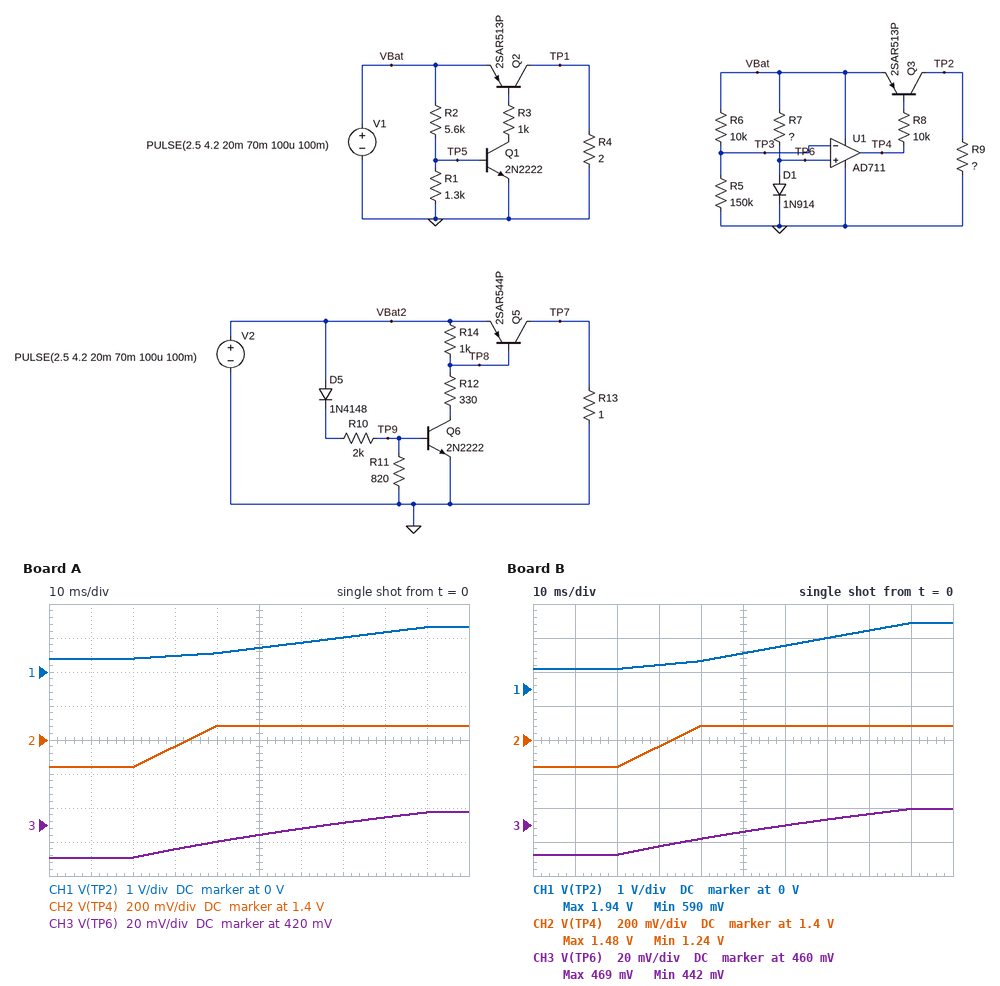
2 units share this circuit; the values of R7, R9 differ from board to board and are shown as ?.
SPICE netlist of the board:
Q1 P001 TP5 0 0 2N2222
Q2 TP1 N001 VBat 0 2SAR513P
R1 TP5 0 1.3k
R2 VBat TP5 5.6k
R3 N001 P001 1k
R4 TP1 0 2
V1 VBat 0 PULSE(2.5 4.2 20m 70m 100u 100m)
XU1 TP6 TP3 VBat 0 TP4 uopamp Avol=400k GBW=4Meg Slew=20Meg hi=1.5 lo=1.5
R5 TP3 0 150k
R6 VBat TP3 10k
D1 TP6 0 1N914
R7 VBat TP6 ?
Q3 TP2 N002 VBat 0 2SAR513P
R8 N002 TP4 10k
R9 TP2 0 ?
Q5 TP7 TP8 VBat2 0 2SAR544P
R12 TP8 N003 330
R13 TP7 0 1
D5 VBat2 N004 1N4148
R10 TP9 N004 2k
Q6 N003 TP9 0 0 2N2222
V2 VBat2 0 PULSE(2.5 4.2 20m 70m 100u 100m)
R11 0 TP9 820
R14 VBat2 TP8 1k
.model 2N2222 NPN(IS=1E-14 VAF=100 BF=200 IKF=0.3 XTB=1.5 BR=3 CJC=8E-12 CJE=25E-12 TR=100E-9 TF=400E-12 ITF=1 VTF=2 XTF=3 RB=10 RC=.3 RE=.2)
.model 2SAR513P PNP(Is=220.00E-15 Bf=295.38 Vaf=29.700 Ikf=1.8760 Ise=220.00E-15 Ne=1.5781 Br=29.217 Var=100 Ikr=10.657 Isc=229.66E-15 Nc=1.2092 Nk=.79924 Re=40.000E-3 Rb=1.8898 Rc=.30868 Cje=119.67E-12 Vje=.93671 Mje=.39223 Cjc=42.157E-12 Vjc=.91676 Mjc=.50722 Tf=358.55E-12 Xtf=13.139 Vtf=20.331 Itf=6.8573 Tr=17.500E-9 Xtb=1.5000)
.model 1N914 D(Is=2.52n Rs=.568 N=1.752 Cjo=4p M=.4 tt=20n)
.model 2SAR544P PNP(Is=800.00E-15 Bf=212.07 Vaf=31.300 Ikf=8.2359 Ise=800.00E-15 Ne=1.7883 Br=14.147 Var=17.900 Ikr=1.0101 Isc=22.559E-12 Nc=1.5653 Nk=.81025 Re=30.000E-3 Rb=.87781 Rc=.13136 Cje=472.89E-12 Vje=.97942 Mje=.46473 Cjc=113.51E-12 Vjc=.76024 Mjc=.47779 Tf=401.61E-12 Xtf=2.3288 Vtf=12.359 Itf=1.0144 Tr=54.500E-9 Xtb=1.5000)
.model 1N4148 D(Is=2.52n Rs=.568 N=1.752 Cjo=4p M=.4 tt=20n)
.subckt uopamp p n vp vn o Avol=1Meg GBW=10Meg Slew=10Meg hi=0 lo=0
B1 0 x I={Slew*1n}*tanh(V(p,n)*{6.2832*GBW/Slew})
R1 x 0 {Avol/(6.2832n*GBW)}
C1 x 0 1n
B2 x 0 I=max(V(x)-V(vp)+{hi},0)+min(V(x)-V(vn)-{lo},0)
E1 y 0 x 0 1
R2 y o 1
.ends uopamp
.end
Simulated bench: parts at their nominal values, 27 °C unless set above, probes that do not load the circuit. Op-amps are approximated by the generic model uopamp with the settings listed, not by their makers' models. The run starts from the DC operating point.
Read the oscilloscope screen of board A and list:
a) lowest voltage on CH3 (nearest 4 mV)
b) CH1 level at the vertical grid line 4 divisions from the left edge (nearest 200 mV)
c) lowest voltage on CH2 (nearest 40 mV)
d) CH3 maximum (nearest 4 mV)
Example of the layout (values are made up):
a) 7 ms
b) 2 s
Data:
a) 400 mV
b) 600 mV
c) 1.24 V
d) 428 mV
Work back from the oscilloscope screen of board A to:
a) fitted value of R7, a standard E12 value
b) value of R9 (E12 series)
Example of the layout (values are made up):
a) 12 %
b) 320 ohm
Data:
a) 120 kΩ
b) 22 Ω
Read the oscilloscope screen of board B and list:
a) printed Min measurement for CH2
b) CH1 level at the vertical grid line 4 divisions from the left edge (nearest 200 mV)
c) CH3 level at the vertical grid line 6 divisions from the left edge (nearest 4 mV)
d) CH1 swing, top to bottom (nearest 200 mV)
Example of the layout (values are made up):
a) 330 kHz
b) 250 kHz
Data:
a) 1.24 V
b) 800 mV
c) 460 mV
d) 1.4 V
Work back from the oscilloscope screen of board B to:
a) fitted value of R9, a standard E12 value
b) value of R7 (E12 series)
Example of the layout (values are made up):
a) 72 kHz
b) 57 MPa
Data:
a) 33 Ω
b) 47 kΩ
